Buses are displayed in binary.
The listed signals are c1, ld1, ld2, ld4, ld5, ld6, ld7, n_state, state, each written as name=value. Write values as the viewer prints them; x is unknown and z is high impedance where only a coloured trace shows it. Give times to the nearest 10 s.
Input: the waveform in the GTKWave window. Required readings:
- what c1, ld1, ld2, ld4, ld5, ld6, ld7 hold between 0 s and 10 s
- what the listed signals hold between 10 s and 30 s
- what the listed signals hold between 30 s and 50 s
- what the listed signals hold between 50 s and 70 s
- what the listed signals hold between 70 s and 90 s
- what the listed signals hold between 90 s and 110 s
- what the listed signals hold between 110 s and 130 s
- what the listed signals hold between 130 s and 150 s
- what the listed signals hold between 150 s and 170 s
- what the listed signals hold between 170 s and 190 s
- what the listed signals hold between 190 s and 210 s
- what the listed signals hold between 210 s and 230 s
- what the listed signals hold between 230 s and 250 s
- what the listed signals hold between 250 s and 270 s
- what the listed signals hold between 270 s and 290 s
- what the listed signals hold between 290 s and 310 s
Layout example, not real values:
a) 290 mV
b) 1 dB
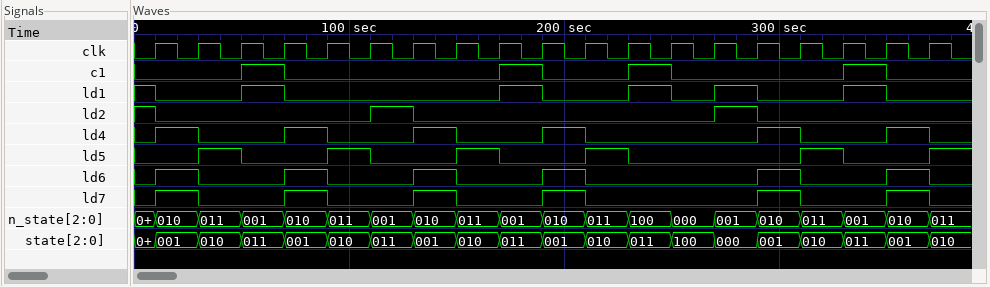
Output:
a) c1=0, ld1=1, ld2=1, ld4=0, ld5=0, ld6=0, ld7=0
b) c1=0, ld1=0, ld2=0, ld4=1, ld5=0, ld6=1, ld7=1, n_state=010, state=001
c) c1=0, ld1=0, ld2=0, ld4=0, ld5=1, ld6=0, ld7=0, n_state=011, state=010
d) c1=1, ld1=1, ld2=0, ld4=0, ld5=0, ld6=0, ld7=0, n_state=001, state=011
e) c1=0, ld1=0, ld2=0, ld4=1, ld5=0, ld6=1, ld7=1, n_state=010, state=001
f) c1=0, ld1=0, ld2=0, ld4=0, ld5=1, ld6=0, ld7=0, n_state=011, state=010
g) c1=0, ld1=0, ld2=1, ld4=0, ld5=0, ld6=0, ld7=0, n_state=001, state=011
h) c1=0, ld1=0, ld2=0, ld4=1, ld5=0, ld6=1, ld7=1, n_state=010, state=001
i) c1=0, ld1=0, ld2=0, ld4=0, ld5=1, ld6=0, ld7=0, n_state=011, state=010
j) c1=1, ld1=1, ld2=0, ld4=0, ld5=0, ld6=0, ld7=0, n_state=001, state=011
k) c1=0, ld1=0, ld2=0, ld4=1, ld5=0, ld6=1, ld7=1, n_state=010, state=001
l) c1=0, ld1=0, ld2=0, ld4=0, ld5=1, ld6=0, ld7=0, n_state=011, state=010
m) c1=1, ld1=1, ld2=0, ld4=0, ld5=0, ld6=0, ld7=0, n_state=100, state=011
n) c1=0, ld1=0, ld2=0, ld4=0, ld5=0, ld6=0, ld7=0, n_state=000, state=100
o) c1=0, ld1=1, ld2=1, ld4=0, ld5=0, ld6=0, ld7=0, n_state=001, state=000
p) c1=0, ld1=0, ld2=0, ld4=1, ld5=0, ld6=1, ld7=1, n_state=010, state=001
